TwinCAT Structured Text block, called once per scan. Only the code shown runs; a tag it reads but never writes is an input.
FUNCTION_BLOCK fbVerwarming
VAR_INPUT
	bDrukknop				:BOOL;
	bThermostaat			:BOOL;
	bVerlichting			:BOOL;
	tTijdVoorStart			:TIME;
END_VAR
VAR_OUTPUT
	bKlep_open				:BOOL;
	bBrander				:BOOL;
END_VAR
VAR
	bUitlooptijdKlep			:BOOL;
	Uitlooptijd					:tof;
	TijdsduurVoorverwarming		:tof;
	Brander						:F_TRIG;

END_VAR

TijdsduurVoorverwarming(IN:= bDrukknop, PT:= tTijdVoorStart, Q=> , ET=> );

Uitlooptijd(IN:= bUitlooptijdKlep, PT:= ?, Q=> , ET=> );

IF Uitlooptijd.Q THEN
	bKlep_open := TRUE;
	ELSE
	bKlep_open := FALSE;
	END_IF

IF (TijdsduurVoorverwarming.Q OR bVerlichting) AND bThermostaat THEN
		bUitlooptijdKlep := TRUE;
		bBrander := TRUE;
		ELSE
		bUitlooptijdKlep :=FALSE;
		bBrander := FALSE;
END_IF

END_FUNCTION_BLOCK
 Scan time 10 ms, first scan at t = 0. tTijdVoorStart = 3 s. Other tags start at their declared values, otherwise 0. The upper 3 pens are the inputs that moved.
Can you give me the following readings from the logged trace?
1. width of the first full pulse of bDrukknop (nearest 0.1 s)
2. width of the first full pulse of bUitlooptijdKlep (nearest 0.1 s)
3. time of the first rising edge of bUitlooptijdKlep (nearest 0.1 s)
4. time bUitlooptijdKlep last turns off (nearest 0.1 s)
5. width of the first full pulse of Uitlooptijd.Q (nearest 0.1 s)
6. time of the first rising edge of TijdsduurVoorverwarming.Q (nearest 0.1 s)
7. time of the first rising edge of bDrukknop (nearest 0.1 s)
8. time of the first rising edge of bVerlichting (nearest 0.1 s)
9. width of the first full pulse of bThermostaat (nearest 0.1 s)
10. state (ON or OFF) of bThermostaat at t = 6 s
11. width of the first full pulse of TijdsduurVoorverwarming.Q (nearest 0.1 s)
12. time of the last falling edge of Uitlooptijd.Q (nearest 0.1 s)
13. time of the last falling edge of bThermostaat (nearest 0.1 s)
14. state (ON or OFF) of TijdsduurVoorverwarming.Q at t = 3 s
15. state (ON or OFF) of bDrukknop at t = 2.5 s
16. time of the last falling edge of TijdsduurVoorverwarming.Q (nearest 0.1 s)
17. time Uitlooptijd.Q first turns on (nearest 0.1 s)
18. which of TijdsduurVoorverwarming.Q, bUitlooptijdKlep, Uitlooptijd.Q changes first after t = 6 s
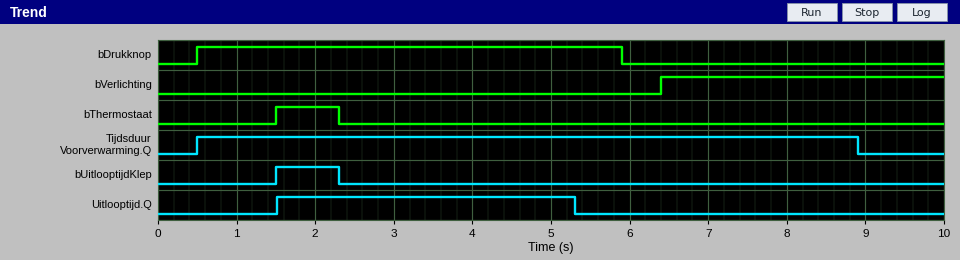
5.4 s
0.8 s
1.5 s
2.3 s
3.8 s
0.5 s
0.5 s
6.4 s
0.8 s
OFF
8.4 s
5.3 s
2.3 s
ON
ON
8.9 s
1.5 s
TijdsduurVoorverwarming.Q
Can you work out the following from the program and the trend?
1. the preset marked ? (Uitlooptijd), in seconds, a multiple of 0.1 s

3.0 s
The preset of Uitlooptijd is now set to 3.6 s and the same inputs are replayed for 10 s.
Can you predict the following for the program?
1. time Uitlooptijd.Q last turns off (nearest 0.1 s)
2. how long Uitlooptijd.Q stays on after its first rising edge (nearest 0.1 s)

5.9 s
4.4 s
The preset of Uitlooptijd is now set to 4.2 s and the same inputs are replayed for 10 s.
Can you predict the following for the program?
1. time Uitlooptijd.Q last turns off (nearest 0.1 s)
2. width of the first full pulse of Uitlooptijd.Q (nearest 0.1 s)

6.5 s
5.0 s
